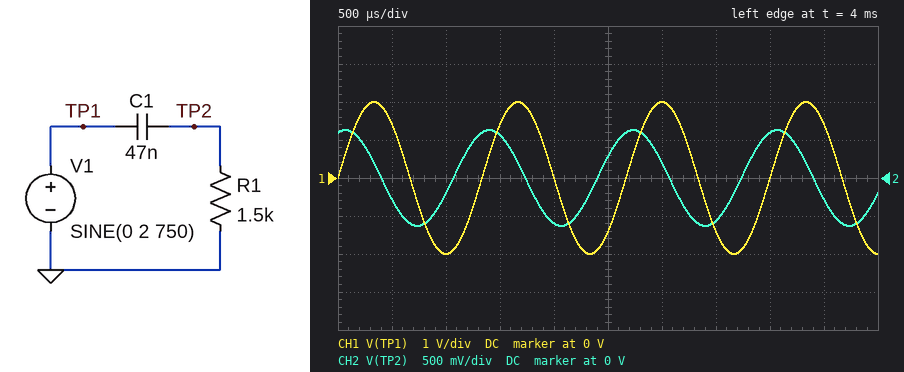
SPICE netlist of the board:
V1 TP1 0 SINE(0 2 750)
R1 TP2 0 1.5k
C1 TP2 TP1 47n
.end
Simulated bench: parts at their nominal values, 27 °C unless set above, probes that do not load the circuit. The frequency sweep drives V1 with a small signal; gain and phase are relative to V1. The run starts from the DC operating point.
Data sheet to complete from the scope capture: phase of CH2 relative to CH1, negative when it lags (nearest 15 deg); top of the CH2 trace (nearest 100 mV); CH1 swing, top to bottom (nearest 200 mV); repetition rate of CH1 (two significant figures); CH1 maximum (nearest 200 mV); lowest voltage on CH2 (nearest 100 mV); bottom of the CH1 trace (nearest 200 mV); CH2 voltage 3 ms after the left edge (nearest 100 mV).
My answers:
75 deg
600 mV
4.0 V
750 Hz
2.0 V
-600 mV
-2.0 V
200 mV
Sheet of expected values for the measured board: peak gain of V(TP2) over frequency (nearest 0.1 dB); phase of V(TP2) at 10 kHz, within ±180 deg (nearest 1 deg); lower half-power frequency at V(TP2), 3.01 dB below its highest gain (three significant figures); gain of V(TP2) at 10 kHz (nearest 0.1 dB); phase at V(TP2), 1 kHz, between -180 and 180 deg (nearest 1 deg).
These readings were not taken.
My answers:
0 dB
13 deg
2.26 kHz
-0.2 dB
66 deg
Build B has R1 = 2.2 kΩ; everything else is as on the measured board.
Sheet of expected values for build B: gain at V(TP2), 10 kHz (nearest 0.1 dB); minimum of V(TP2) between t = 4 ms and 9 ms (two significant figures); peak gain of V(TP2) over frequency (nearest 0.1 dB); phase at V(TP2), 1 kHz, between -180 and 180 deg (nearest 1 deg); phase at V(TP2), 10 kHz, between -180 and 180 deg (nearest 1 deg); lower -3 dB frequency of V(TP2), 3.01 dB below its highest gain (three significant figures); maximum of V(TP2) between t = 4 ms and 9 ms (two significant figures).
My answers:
-0.1 dB
-880 mV
0 dB
57 deg
9 deg
1.54 kHz
880 mV
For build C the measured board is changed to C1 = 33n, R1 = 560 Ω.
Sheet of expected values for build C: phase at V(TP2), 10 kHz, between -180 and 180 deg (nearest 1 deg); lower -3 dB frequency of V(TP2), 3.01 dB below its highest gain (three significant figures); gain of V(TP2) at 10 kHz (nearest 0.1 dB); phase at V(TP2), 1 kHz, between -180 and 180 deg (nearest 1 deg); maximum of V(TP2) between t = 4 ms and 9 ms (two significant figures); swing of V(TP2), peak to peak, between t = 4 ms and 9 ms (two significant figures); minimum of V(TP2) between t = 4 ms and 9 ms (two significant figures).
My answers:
41 deg
8.61 kHz
-2.4 dB
83 deg
170 mV
350 mV
-170 mV
